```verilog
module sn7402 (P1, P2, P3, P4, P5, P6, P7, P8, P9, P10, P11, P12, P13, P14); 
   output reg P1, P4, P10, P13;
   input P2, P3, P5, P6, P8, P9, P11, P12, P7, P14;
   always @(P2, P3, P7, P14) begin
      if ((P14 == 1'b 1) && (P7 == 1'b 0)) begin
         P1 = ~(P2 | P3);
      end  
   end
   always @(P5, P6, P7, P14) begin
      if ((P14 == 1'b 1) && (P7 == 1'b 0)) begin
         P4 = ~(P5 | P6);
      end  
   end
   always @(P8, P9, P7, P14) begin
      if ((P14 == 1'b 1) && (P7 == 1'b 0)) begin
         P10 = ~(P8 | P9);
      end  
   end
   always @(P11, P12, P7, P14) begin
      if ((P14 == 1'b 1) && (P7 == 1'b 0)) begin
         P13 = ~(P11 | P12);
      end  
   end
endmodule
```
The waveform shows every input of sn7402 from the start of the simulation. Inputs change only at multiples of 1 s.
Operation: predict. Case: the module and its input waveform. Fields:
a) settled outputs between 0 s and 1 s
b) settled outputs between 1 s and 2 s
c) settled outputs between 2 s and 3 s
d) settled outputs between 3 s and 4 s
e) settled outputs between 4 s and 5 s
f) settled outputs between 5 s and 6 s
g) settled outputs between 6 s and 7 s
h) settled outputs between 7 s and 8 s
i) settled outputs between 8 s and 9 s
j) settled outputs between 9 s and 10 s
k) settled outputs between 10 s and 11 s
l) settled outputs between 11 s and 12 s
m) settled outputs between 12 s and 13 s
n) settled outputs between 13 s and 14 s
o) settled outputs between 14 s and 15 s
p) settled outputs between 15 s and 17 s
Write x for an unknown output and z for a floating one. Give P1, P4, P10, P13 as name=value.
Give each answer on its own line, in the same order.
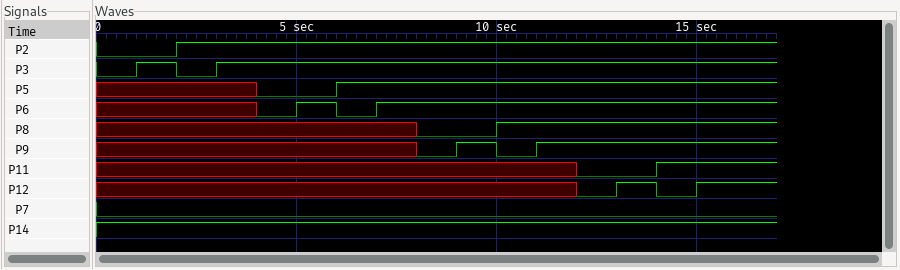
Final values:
P1=1, P4=x, P10=x, P13=x
P1=0, P4=x, P10=x, P13=x
P1=0, P4=x, P10=x, P13=x
P1=0, P4=x, P10=x, P13=x
P1=0, P4=1, P10=x, P13=x
P1=0, P4=0, P10=x, P13=x
P1=0, P4=0, P10=x, P13=x
P1=0, P4=0, P10=x, P13=x
P1=0, P4=0, P10=1, P13=x
P1=0, P4=0, P10=0, P13=x
P1=0, P4=0, P10=0, P13=x
P1=0, P4=0, P10=0, P13=x
P1=0, P4=0, P10=0, P13=1
P1=0, P4=0, P10=0, P13=0
P1=0, P4=0, P10=0, P13=0
P1=0, P4=0, P10=0, P13=0
